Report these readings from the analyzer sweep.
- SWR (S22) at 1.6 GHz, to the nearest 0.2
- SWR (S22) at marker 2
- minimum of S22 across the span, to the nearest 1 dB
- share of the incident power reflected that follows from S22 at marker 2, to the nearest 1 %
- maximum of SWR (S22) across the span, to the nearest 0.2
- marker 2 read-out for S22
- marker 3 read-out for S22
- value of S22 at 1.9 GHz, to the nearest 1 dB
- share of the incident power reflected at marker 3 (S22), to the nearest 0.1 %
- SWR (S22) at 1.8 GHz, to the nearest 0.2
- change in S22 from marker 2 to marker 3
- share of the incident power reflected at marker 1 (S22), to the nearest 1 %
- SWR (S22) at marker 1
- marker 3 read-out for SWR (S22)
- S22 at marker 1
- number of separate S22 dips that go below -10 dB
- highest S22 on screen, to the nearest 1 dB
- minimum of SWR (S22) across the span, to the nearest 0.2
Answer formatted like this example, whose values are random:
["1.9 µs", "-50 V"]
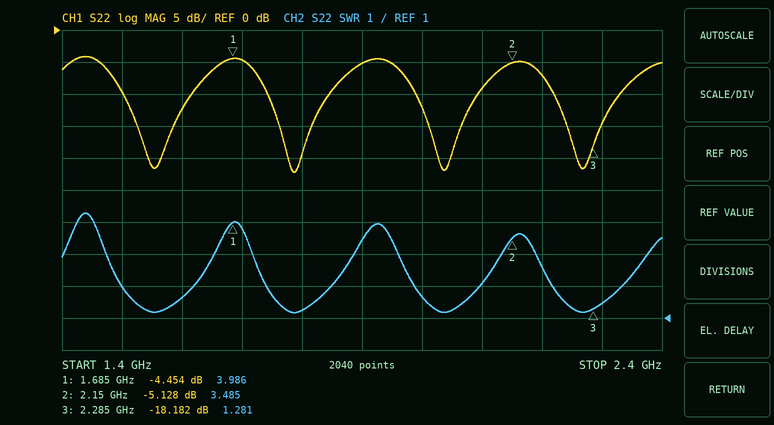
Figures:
["1.6", "3.485", "-22 dB", "31 %", "4.2", "-5.128 dB", "-18.182 dB", "-5 dB", "1.5 %", "1.2", "-13.054 dB", "36 %", "3.986", "1.281", "-4.454 dB", "4", "-4 dB", "1.2"]
